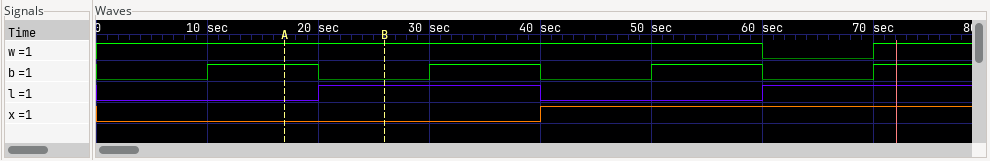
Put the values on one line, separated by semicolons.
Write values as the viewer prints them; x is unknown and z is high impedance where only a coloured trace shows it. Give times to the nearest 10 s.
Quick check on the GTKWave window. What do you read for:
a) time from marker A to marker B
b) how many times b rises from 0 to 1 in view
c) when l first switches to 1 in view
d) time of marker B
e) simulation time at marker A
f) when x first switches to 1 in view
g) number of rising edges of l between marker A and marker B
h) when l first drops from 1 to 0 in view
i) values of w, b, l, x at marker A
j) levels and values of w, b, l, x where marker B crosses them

10 s; 4; 20 s; 30 s; 20 s; 40 s; 1; 40 s; w=1, b=1, l=0, x=0; w=1, b=0, l=1, x=0
